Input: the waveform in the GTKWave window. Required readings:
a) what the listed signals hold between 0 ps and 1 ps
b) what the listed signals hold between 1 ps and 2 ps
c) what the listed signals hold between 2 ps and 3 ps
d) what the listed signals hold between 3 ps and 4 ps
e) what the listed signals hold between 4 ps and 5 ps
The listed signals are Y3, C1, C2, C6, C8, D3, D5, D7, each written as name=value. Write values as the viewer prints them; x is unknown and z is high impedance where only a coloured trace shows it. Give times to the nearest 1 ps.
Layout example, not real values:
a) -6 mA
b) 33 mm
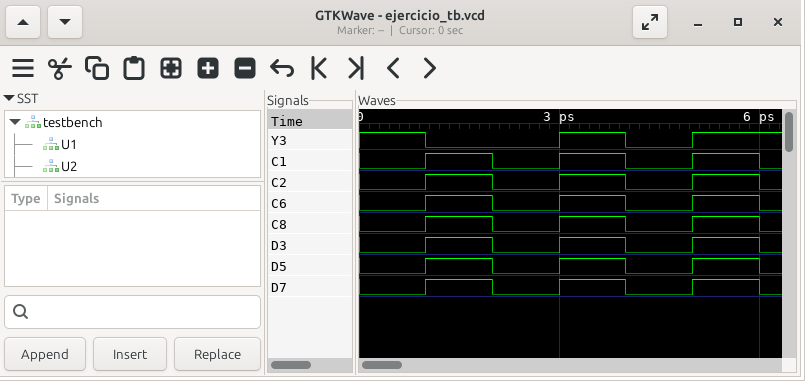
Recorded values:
a) Y3=1, C1=0, C2=0, C6=0, C8=0, D3=0, D5=0, D7=0
b) Y3=0, C1=1, C2=1, C6=1, C8=1, D3=1, D5=1, D7=1
c) Y3=0, C1=0, C2=0, C6=0, C8=0, D3=0, D5=0, D7=0
d) Y3=1, C1=1, C2=1, C6=1, C8=1, D3=1, D5=1, D7=1
e) Y3=0, C1=0, C2=0, C6=0, C8=0, D3=0, D5=0, D7=0
